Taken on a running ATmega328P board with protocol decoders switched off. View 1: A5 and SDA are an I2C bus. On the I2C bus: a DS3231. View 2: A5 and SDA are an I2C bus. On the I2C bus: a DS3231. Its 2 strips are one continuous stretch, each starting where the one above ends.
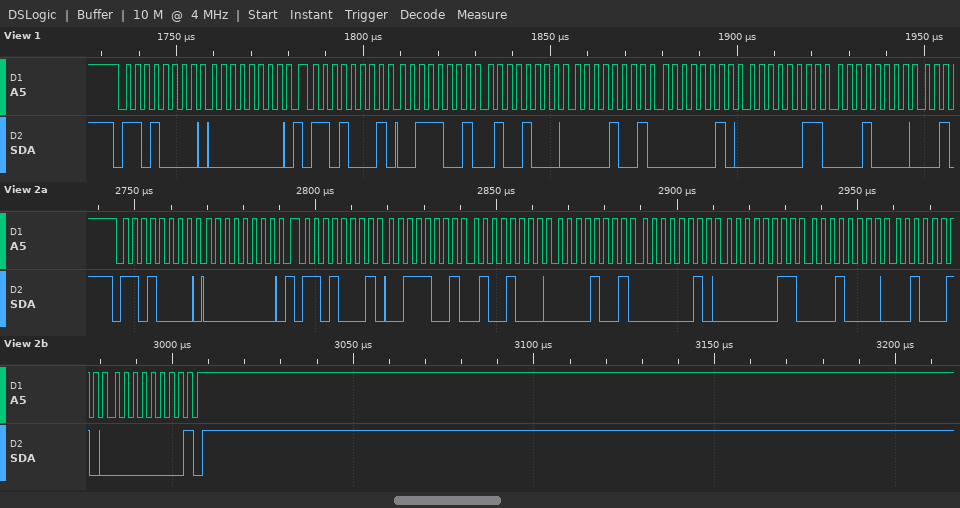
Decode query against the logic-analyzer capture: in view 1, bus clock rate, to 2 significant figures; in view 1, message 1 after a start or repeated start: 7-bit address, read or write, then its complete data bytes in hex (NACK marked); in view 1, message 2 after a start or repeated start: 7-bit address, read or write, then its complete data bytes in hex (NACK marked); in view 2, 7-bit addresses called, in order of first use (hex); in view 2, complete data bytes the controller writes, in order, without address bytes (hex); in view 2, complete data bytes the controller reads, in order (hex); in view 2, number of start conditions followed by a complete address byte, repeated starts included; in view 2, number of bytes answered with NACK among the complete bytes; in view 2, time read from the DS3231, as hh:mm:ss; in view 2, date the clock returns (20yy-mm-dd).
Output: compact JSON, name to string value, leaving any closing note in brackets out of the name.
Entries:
{"in view 1, bus clock rate, to 2 significant figures": "400 kHz", "in view 1, message 1 after a start or repeated start: 7-bit address, read or write, then its complete data bytes in hex": "0x68 write: 00", "in view 1, message 2 after a start or repeated start: 7-bit address, read or write, then its complete data bytes in hex": "0x68 read: 39 48 09 02 03 10", "in view 2, 7-bit addresses called, in order of first use": "0x68", "in view 2, complete data bytes the controller writes, in order, without address bytes": "00", "in view 2, complete data bytes the controller reads, in order": "39 48 09 02 03 10 22 00", "in view 2, number of start conditions followed by a complete address byte, repeated starts included": "2", "in view 2, number of bytes answered with NACK among the complete bytes": "1", "in view 2, time read from the DS3231, as hh:mm:ss": "09:48:39", "in view 2, date the clock returns": "2022-10-03"}
